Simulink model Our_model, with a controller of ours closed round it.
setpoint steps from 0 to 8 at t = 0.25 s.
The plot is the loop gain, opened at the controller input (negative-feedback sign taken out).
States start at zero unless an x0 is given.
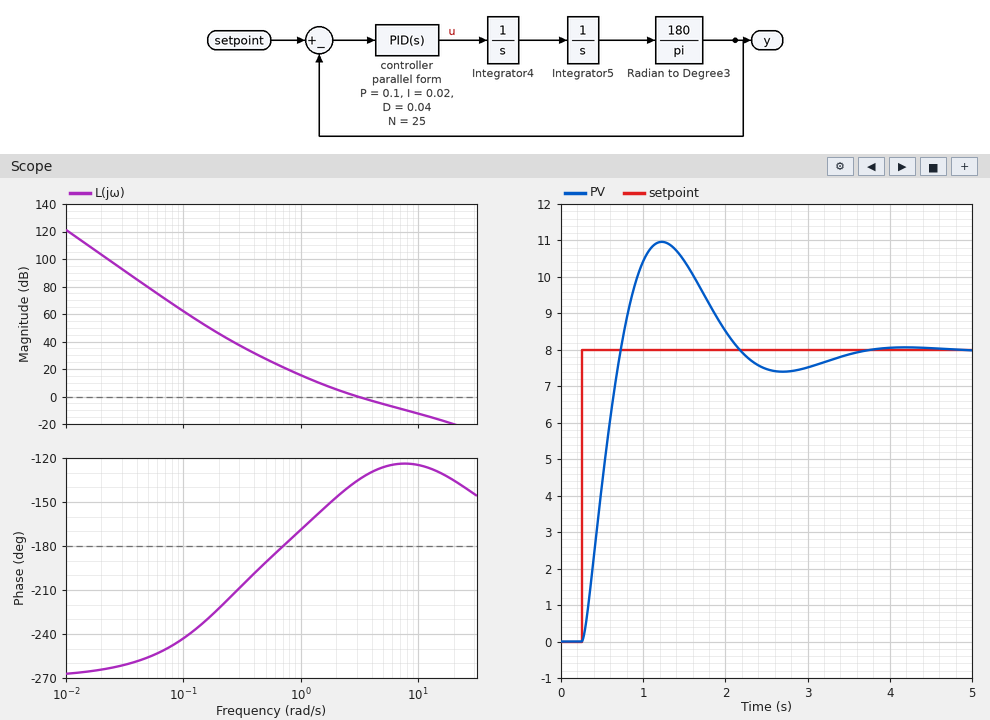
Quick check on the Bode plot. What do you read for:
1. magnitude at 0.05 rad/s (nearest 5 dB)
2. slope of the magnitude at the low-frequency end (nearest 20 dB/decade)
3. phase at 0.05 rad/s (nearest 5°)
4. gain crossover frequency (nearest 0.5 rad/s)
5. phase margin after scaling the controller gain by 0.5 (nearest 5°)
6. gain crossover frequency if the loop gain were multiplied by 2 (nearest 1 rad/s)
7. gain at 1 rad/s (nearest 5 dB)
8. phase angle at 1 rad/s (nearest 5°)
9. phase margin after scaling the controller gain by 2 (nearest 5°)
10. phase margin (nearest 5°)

80 dB
-60 dB/decade
-255°
3.0 rad/s
30°
5 rad/s
15 dB
-170°
55°
45°
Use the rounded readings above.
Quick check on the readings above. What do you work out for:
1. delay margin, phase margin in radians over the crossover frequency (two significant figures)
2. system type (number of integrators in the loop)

0.26 s
3
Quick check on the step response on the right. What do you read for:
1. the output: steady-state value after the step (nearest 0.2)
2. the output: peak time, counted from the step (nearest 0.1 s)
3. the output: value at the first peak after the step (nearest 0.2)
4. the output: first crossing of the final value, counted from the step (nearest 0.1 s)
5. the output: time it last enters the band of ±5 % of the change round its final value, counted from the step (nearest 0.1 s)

8.0
1.0 s
11.0
0.5 s
2.9 s
